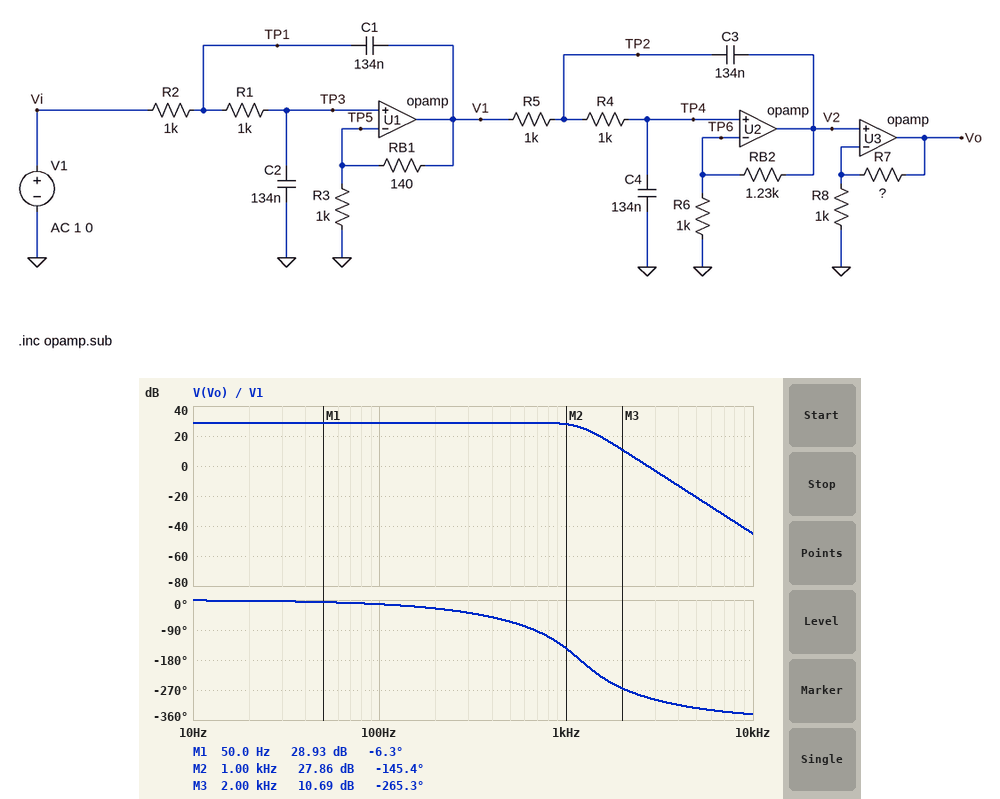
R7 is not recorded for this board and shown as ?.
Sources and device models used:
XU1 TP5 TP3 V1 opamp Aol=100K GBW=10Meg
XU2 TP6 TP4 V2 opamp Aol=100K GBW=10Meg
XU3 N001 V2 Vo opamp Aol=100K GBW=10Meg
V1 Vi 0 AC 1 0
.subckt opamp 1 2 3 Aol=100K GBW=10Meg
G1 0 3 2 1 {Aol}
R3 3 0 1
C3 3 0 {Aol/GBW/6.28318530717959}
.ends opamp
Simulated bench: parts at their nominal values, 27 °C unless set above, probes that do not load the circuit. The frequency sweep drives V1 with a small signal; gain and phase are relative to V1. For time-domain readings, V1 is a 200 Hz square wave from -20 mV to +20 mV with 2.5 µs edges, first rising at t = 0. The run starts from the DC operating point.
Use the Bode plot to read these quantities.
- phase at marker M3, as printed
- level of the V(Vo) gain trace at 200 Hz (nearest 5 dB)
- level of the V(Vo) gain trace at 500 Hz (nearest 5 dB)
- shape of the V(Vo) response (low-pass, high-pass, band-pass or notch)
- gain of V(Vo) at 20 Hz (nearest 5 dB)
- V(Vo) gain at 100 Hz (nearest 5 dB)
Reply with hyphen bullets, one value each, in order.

- -265.3 deg
- 30 dB
- 30 dB
- low-pass
- 30 dB
- 30 dB
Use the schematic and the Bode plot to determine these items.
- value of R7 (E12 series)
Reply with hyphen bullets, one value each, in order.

- 10 kΩ
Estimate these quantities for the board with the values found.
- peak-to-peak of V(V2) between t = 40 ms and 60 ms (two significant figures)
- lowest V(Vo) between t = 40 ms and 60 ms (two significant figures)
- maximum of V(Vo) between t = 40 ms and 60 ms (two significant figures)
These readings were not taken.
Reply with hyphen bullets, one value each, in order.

- 120 mV
- -680 mV
- 680 mV
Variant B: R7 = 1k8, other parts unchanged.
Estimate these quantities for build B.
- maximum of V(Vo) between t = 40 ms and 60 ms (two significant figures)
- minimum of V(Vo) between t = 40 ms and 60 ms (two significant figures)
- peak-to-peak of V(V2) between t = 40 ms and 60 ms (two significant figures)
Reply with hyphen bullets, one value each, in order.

- 170 mV
- -170 mV
- 120 mV
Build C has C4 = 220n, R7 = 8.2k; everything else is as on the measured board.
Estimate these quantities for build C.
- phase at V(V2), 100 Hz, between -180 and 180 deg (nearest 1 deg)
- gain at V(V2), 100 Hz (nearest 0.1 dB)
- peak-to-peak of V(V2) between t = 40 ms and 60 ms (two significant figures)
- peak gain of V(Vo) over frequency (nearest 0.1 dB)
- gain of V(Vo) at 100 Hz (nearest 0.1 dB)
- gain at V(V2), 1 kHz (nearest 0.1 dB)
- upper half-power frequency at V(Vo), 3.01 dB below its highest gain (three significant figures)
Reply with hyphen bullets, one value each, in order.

- -19 deg
- 8.0 dB
- 100 mV
- 27.4 dB
- 27.3 dB
- -0.7 dB
- 594 Hz
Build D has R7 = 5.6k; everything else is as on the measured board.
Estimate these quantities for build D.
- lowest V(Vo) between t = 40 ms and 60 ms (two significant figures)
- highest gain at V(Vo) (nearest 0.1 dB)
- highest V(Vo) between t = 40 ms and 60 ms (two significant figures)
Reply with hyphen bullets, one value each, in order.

- -410 mV
- 24.5 dB
- 410 mV
